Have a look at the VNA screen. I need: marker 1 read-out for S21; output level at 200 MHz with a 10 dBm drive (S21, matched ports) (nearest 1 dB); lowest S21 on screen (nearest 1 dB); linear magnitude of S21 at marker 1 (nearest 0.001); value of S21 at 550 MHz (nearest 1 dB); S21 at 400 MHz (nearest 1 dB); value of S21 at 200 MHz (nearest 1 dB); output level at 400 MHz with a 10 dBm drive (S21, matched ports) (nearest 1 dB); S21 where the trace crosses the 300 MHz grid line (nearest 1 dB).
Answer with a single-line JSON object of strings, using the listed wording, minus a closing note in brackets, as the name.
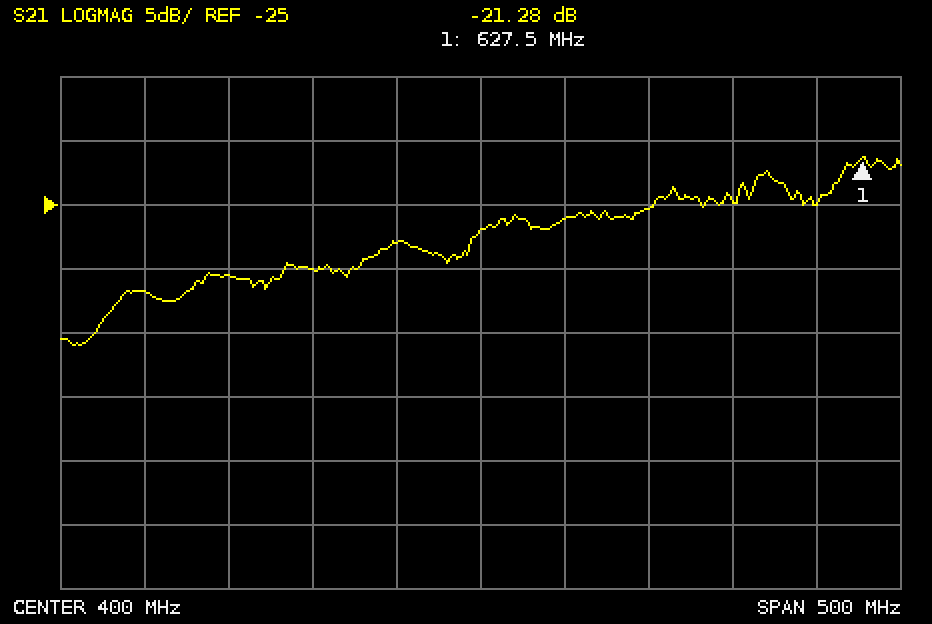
{"marker 1 read-out for S21": "-21.28 dB", "output level at 200 MHz with a 10 dBm drive (S21, matched ports)": "-22 dBm", "lowest S21 on screen": "-36 dB", "linear magnitude of S21 at marker 1": "0.086", "value of S21 at 550 MHz": "-25 dB", "S21 at 400 MHz": "-27 dB", "value of S21 at 200 MHz": "-32 dB", "output level at 400 MHz with a 10 dBm drive (S21, matched ports)": "-17 dBm", "S21 where the trace crosses the 300 MHz grid line": "-30 dB"}
